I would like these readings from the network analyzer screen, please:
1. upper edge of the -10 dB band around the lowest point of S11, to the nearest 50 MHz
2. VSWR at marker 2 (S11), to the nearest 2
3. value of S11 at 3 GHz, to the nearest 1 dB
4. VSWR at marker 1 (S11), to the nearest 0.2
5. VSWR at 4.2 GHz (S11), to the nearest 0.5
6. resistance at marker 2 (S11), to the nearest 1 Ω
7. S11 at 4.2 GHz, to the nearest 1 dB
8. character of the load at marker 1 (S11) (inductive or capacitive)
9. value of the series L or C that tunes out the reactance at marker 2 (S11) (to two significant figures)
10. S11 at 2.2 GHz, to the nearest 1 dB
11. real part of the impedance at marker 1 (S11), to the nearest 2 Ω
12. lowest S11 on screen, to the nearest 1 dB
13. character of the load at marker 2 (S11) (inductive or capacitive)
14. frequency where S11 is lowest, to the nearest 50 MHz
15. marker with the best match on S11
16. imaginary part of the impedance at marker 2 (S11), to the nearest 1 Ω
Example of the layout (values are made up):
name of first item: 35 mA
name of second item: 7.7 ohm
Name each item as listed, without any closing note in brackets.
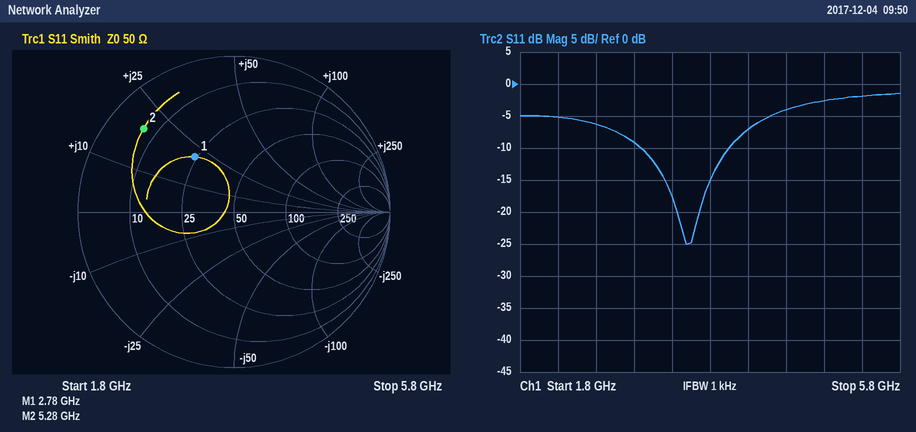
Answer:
upper edge of the -10 dB band around the lowest point of S11, to the nearest 50 MHz: 4.00 GHz
VSWR at marker 2 (S11), to the nearest 2: 8
value of S11 at 3 GHz, to the nearest 1 dB: -9 dB
VSWR at marker 1 (S11), to the nearest 0.2: 2.6
VSWR at 4.2 GHz (S11), to the nearest 0.5: 2.5
resistance at marker 2 (S11), to the nearest 1 Ω: 7 Ω
S11 at 4.2 GHz, to the nearest 1 dB: -7 dB
character of the load at marker 1 (S11): inductive
value of the series L or C that tunes out the reactance at marker 2 (S11): 1.6 pF
S11 at 2.2 GHz, to the nearest 1 dB: -5 dB
real part of the impedance at marker 1 (S11), to the nearest 2 Ω: 24 Ω
lowest S11 on screen, to the nearest 1 dB: -25 dB
character of the load at marker 2 (S11): inductive
frequency where S11 is lowest, to the nearest 50 MHz: 3.55 GHz
marker with the best match on S11: marker 1
imaginary part of the impedance at marker 2 (S11), to the nearest 1 Ω: +19 Ω
